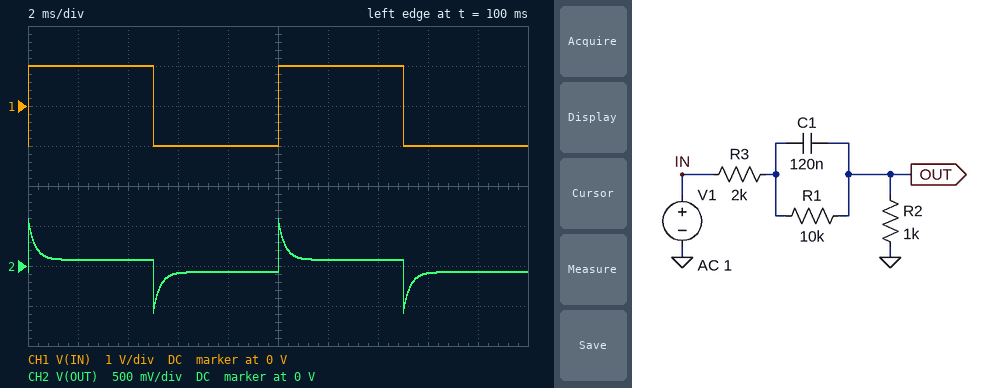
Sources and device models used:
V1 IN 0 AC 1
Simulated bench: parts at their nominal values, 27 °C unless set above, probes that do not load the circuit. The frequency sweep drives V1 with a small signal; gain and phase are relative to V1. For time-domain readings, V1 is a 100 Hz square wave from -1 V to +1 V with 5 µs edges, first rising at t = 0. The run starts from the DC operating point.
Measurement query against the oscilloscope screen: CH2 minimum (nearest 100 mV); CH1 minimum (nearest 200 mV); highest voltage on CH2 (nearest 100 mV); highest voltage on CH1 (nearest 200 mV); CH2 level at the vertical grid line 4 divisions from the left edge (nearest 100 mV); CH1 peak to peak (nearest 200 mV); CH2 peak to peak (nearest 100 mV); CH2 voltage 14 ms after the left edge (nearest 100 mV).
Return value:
-600 mV
-1.0 V
600 mV
1.0 V
-100 mV
2.0 V
1.2 V
100 mV
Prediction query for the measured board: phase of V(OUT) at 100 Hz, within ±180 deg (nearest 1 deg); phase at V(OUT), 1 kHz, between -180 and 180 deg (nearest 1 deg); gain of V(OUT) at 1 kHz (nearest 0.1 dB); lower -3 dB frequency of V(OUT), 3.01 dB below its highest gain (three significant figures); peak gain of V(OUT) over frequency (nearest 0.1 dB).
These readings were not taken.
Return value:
27 deg
22 deg
-10.7 dB
543 Hz
-9.5 dB
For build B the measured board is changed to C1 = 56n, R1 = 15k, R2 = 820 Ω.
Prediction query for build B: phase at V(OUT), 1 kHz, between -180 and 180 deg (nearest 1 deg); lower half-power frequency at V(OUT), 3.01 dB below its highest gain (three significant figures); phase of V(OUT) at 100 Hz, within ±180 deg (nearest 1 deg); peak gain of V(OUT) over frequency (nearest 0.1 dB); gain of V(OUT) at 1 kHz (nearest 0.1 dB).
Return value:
39 deg
1.17 kHz
23 deg
-10.7 dB
-14.4 dB
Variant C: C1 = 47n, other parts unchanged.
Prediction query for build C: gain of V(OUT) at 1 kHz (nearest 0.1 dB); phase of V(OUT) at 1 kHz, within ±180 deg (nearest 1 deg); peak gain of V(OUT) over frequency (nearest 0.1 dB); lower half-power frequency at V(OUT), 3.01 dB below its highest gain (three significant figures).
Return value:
-14.1 dB
37 deg
-9.5 dB
1.39 kHz
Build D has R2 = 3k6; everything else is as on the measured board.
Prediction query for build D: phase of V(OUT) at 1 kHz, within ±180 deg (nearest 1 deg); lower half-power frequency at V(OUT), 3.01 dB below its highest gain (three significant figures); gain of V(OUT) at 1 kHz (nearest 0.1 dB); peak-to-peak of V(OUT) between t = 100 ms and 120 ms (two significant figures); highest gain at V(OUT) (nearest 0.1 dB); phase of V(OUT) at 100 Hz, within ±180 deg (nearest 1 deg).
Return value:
13 deg
318 Hz
-4.3 dB
2.1 V
-3.8 dB
22 deg
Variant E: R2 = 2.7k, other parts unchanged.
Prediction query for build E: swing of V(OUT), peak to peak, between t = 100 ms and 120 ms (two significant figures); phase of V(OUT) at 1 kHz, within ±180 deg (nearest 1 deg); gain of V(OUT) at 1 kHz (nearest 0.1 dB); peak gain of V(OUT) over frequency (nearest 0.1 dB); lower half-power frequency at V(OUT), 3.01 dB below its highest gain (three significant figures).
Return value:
1.9 V
15 deg
-5.4 dB
-4.8 dB
370 Hz
